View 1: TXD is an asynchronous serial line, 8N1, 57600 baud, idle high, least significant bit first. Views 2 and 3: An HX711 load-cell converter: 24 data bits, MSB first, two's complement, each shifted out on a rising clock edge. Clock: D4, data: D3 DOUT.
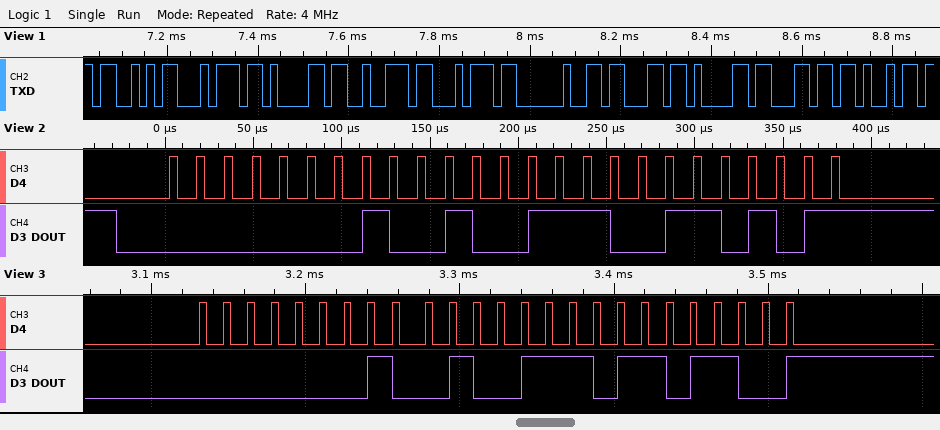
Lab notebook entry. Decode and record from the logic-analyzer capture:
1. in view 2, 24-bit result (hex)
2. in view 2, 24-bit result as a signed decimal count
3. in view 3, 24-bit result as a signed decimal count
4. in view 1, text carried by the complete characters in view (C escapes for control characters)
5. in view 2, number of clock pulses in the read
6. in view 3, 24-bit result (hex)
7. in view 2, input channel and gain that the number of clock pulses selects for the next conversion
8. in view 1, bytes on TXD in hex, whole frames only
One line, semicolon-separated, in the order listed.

0x012735; 75573; 75628; "Start cali"; 25; 0x01276C; channel A, gain 128; 0x53 0x74 0x61 0x72 0x74 0x20 0x63 0x61 0x6C 0x69
